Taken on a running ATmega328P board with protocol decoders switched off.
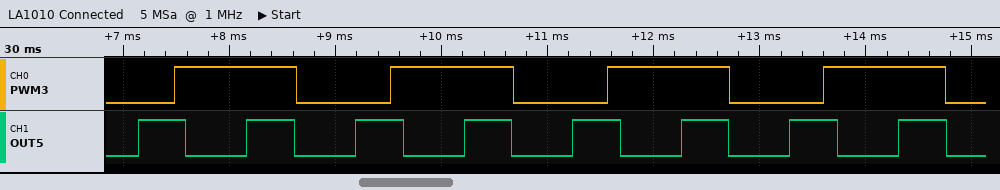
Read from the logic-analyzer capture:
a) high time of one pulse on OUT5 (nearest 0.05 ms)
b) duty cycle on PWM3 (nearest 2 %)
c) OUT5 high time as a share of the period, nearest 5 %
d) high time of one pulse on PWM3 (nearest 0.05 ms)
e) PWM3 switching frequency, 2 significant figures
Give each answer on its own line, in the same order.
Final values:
0.45 ms
56 %
45 %
1.15 ms
490 Hz
